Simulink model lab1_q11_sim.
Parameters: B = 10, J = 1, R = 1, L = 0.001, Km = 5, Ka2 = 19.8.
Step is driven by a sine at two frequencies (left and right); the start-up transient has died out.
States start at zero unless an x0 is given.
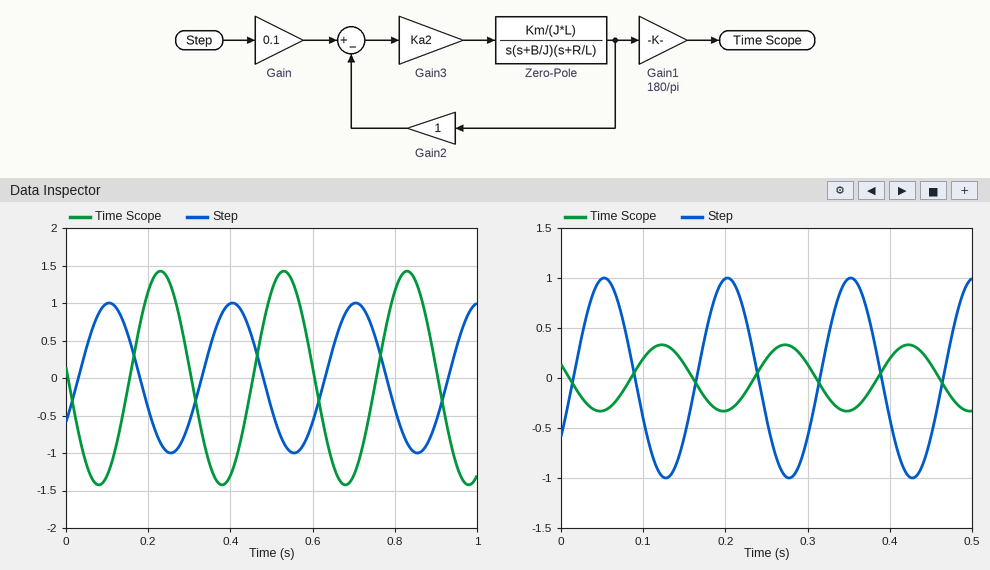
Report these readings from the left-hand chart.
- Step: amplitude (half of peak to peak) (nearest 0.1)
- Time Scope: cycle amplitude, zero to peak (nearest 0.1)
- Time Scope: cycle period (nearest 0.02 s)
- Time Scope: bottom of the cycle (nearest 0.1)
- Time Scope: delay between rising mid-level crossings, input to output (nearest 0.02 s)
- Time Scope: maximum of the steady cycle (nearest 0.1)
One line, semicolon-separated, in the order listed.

1.0; 1.4; 0.30 s; -1.4; 0.12 s; 1.4
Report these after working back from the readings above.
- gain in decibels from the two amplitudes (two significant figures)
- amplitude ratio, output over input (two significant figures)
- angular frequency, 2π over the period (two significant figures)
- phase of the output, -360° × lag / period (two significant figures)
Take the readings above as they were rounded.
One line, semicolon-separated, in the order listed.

2.9 dB; 1.4; 21 rad/s; -140°
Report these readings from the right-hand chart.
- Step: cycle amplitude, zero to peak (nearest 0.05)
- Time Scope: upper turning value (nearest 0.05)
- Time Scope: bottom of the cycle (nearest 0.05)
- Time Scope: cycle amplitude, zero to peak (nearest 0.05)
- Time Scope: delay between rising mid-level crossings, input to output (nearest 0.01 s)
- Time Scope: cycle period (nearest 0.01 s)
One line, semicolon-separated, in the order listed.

1.00; 0.35; -0.35; 0.35; 0.07 s; 0.15 s
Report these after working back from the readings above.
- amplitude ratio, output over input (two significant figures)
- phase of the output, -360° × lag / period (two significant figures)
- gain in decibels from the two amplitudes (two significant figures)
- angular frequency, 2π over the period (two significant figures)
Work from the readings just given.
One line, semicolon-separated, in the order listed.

0.35; -170°; -9.1 dB; 42 rad/s
